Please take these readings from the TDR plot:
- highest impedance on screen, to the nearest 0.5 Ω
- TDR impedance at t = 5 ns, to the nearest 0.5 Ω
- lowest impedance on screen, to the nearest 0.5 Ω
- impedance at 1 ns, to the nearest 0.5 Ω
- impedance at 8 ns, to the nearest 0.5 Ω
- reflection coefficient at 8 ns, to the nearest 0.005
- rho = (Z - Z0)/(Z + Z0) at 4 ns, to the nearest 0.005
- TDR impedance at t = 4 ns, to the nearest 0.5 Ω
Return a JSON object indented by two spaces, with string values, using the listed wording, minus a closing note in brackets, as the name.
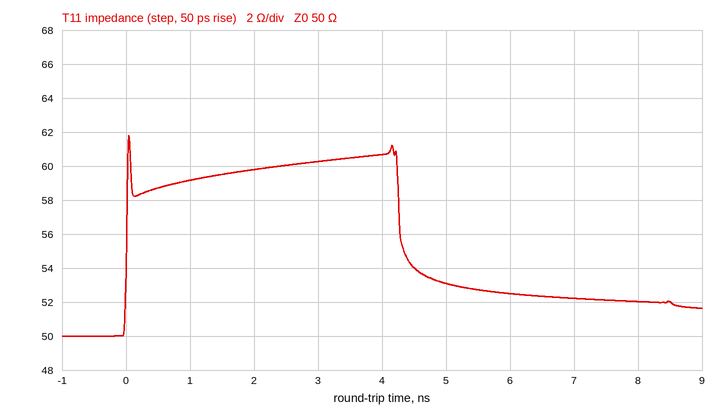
{
  "highest impedance on screen, to the nearest 0.5 Ω": "62.0 Ω",
  "TDR impedance at t = 5 ns, to the nearest 0.5 Ω": "53.0 Ω",
  "lowest impedance on screen, to the nearest 0.5 Ω": "50.0 Ω",
  "impedance at 1 ns, to the nearest 0.5 Ω": "59.0 Ω",
  "impedance at 8 ns, to the nearest 0.5 Ω": "52.0 Ω",
  "reflection coefficient at 8 ns, to the nearest 0.005": "+0.020",
  "rho = (Z - Z0)/(Z + Z0) at 4 ns, to the nearest 0.005": "+0.095",
  "TDR impedance at t = 4 ns, to the nearest 0.5 Ω": "60.5 Ω"
}
